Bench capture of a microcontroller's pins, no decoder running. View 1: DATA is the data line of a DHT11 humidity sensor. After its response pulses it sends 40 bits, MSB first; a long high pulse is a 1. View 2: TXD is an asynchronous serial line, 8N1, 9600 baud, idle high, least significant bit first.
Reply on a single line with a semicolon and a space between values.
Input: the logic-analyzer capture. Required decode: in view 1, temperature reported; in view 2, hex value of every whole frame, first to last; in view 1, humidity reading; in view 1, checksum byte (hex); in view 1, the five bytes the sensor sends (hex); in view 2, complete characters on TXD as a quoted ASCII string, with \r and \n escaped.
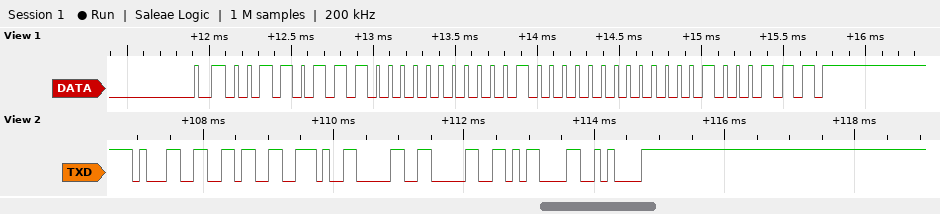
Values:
16.0 °C; 0x31 0x36 0x2E 0x30 0x30 0x0D 0x0A; 55 %; 0x47; 37 00 10 00 47; "16.00\r\n"
